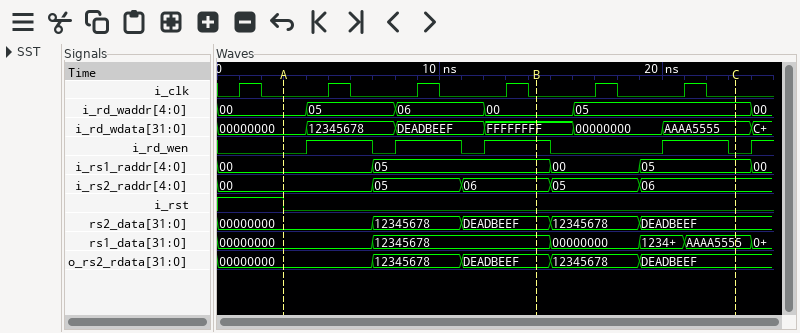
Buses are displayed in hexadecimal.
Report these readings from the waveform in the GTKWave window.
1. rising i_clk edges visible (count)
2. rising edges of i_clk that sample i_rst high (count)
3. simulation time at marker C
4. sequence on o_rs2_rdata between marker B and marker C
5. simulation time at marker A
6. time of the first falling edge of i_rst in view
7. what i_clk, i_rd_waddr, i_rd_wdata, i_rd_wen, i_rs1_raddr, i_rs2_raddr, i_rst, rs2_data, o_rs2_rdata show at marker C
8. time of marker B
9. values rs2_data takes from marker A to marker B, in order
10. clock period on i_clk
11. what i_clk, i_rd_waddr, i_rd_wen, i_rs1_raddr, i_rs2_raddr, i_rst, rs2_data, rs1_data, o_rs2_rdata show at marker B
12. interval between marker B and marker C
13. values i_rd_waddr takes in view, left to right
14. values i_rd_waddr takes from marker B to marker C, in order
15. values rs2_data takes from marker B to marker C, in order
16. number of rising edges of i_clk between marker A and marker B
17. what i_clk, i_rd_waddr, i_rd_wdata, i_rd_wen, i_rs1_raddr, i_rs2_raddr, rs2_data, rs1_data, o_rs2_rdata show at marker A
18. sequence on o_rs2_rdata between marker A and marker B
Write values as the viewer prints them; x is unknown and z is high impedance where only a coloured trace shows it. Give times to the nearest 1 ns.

6
1
23 ns
DEADBEEF, 12345678, DEADBEEF
3 ns
3 ns
i_clk=0, i_rd_waddr=05, i_rd_wdata=AAAA5555, i_rd_wen=0, i_rs1_raddr=05, i_rs2_raddr=06, i_rst=0, rs2_data=DEADBEEF, o_rs2_rdata=DEADBEEF
14 ns
00000000, 12345678, DEADBEEF
4 ns
i_clk=0, i_rd_waddr=00, i_rd_wen=1, i_rs1_raddr=05, i_rs2_raddr=06, i_rst=0, rs2_data=DEADBEEF, rs1_data=12345678, o_rs2_rdata=DEADBEEF
9 ns
00, 05, 06, 00, 05, 00
00, 05
DEADBEEF, 12345678, DEADBEEF
3
i_clk=0, i_rd_waddr=00, i_rd_wdata=00000000, i_rd_wen=0, i_rs1_raddr=00, i_rs2_raddr=00, rs2_data=00000000, rs1_data=00000000, o_rs2_rdata=00000000
00000000, 12345678, DEADBEEF
